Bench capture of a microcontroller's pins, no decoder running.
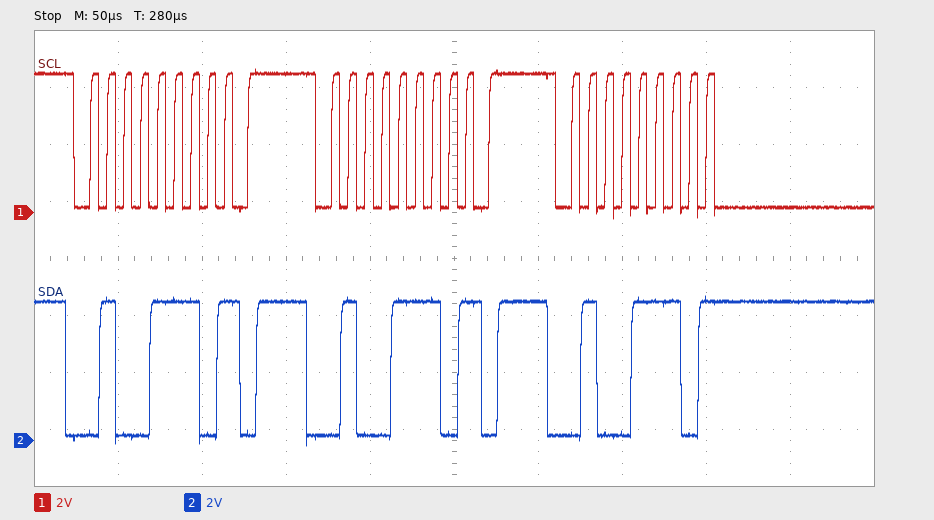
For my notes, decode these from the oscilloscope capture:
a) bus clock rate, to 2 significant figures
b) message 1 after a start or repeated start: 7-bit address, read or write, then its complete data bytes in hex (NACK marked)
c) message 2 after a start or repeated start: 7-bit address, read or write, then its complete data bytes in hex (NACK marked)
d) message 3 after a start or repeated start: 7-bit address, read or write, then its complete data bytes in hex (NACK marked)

100 kHz
0x27 write NACK
0x27 write NACK
0x27 write NACK
